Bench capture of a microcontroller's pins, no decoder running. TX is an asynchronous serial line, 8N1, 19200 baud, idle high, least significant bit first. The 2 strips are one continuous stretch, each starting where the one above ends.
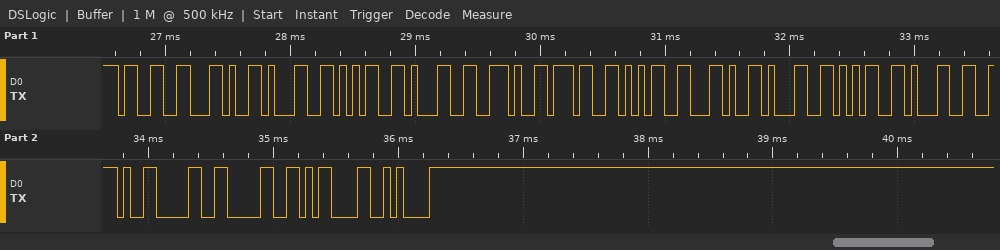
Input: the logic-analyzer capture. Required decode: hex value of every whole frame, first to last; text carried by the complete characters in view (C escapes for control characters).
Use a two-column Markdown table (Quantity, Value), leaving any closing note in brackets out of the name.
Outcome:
| Quantity | Value |
|---|---|
| hex value of every whole frame, first to last | 33 2C 31 35 31 2E 37 35 2C 31 35 31 2E 30 30 0D 0A |
| text carried by the complete characters in view | "3,151.75,151.00\r\n" |
